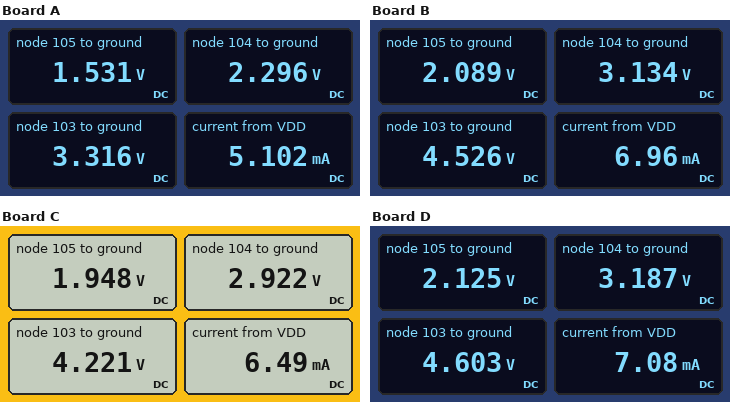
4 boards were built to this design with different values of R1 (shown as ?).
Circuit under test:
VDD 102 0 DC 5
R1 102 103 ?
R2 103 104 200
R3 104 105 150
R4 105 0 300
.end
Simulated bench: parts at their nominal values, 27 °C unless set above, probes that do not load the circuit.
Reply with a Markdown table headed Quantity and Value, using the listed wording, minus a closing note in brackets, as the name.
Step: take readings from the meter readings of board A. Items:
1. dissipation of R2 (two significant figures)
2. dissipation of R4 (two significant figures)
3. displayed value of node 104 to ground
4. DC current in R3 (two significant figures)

| Quantity | Value |
|---|---|
| dissipation of R2 | 5.2 mW |
| dissipation of R4 | 7.8 mW |
| displayed value of node 104 to ground | 2.296 V |
| DC current in R3 | 5.1 mA |
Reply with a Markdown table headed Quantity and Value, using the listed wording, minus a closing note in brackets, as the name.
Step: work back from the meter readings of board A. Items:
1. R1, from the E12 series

| Quantity | Value |
|---|---|
| R1, from the E12 series | 330 Ω |
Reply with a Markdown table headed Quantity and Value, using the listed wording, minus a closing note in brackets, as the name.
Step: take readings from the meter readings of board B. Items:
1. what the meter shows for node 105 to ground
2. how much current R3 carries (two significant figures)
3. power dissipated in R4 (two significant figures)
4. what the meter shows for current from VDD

| Quantity | Value |
|---|---|
| what the meter shows for node 105 to ground | 2.089 V |
| how much current R3 carries | 7.0 mA |
| power dissipated in R4 | 15 mW |
| what the meter shows for current from VDD | 6.96 mA |
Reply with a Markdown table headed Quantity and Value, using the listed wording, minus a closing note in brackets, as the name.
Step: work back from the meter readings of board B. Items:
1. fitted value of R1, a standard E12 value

| Quantity | Value |
|---|---|
| fitted value of R1, a standard E12 value | 68 Ω |
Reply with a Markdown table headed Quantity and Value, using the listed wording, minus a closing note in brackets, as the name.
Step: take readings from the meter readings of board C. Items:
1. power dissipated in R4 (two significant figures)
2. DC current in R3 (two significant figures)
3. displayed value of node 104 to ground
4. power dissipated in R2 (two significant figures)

| Quantity | Value |
|---|---|
| power dissipated in R4 | 13 mW |
| DC current in R3 | 6.5 mA |
| displayed value of node 104 to ground | 2.922 V |
| power dissipated in R2 | 8.4 mW |
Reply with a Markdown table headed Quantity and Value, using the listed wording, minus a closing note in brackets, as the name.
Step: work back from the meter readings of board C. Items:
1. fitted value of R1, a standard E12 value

| Quantity | Value |
|---|---|
| fitted value of R1, a standard E12 value | 120 Ω |
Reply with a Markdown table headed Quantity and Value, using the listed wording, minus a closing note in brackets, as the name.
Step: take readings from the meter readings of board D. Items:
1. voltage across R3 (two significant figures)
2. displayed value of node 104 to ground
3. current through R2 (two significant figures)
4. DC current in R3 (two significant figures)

| Quantity | Value |
|---|---|
| voltage across R3 | 1.1 V |
| displayed value of node 104 to ground | 3.187 V |
| current through R2 | 7.1 mA |
| DC current in R3 | 7.1 mA |
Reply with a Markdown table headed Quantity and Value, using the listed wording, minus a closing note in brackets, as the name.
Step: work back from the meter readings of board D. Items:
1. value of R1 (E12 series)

| Quantity | Value |
|---|---|
| value of R1 | 56 Ω |
